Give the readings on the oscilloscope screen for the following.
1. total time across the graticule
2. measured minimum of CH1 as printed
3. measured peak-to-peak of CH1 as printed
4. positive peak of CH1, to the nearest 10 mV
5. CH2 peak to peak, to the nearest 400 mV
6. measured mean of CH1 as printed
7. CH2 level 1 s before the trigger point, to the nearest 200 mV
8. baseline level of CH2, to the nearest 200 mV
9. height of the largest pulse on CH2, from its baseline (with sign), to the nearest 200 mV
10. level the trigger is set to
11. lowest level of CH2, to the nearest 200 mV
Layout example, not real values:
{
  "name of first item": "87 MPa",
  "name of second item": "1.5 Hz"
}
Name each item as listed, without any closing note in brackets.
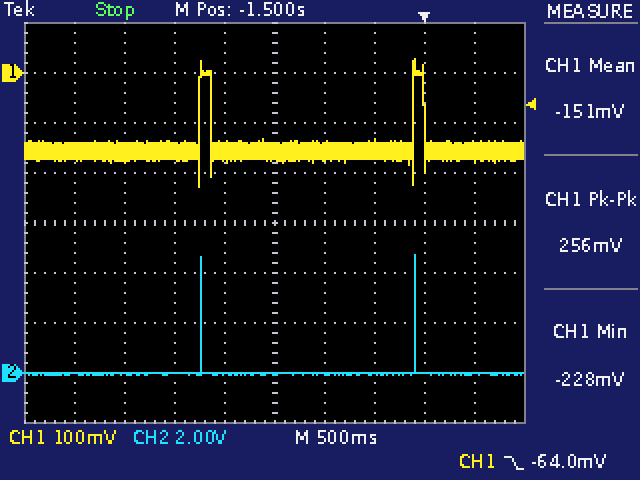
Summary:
{
  "total time across the graticule": "5 s",
  "measured minimum of CH1 as printed": "-228 mV",
  "measured peak-to-peak of CH1 as printed": "256 mV",
  "positive peak of CH1, to the nearest 10 mV": "30 mV",
  "CH2 peak to peak, to the nearest 400 mV": "4.8 V",
  "measured mean of CH1 as printed": "-151 mV",
  "CH2 level 1 s before the trigger point, to the nearest 200 mV": "0.0 V",
  "baseline level of CH2, to the nearest 200 mV": "0.0 V",
  "height of the largest pulse on CH2, from its baseline (with sign), to the nearest 200 mV": "+4.8 V",
  "level the trigger is set to": "-64.0 mV",
  "lowest level of CH2, to the nearest 200 mV": "0.0 V"
}
